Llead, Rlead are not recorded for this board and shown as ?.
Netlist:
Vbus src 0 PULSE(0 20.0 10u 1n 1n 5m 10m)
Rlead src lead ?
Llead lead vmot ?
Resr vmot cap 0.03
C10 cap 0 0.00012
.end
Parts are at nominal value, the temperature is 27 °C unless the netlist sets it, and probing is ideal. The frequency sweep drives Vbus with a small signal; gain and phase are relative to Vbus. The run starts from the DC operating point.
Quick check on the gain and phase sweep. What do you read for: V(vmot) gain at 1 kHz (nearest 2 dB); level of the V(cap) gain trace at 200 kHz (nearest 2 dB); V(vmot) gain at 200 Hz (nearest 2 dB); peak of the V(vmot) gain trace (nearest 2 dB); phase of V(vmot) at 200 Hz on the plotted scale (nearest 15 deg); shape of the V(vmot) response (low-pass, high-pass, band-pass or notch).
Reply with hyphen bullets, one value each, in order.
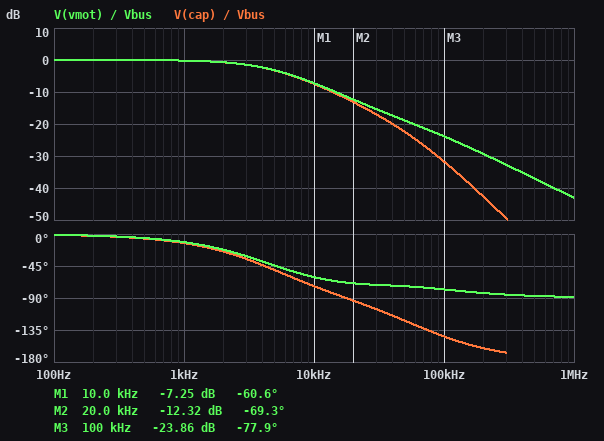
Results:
- 0 dB
- -42 dB
- 0 dB
- 0 dB
- 0 deg
- low-pass
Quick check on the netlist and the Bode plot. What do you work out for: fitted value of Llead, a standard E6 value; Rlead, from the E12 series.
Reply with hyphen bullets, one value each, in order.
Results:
- 680 nH
- 0.27 Ω
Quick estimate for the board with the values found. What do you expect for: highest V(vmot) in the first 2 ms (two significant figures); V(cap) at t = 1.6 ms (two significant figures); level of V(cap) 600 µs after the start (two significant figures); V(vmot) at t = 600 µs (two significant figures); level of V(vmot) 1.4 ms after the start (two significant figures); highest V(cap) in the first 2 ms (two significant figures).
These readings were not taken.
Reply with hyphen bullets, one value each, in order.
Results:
- 20 V
- 20 V
- 20 V
- 20 V
- 20 V
- 20 V
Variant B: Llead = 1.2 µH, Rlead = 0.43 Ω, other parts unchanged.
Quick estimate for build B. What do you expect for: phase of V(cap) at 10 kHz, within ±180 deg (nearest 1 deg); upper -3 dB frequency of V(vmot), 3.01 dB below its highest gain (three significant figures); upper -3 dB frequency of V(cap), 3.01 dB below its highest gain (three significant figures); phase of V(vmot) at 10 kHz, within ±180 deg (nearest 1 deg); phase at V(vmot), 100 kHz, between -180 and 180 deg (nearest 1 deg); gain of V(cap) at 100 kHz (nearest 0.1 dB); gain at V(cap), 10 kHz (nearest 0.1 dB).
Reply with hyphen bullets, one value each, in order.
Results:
- -83 deg
- 3.04 kHz
- 3.03 kHz
- -70 deg
- -82 deg
- -36.4 dB
- -10.9 dB
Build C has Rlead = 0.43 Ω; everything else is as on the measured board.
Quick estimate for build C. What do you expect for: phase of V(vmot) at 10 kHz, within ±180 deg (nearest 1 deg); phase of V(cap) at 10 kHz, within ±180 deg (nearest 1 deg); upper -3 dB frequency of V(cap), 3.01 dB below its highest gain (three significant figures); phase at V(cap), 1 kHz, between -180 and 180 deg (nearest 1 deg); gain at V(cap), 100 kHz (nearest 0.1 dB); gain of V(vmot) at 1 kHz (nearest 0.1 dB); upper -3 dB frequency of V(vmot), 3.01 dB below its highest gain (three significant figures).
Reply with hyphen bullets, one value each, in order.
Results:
- -66 deg
- -79 deg
- 2.96 kHz
- -19 deg
- -33.4 dB
- -0.5 dB
- 2.98 kHz
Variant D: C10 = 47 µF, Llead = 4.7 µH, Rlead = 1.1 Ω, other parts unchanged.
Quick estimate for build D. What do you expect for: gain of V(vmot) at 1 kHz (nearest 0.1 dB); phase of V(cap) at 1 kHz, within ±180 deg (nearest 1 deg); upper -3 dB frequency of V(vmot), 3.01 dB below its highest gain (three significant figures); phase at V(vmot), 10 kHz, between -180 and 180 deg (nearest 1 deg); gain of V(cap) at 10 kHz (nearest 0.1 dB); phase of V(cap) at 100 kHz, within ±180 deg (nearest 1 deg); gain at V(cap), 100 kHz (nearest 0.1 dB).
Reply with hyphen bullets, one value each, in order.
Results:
- -0.4 dB
- -19 deg
- 3.25 kHz
- -83 deg
- -10.5 dB
- -159 deg
- -39.3 dB
